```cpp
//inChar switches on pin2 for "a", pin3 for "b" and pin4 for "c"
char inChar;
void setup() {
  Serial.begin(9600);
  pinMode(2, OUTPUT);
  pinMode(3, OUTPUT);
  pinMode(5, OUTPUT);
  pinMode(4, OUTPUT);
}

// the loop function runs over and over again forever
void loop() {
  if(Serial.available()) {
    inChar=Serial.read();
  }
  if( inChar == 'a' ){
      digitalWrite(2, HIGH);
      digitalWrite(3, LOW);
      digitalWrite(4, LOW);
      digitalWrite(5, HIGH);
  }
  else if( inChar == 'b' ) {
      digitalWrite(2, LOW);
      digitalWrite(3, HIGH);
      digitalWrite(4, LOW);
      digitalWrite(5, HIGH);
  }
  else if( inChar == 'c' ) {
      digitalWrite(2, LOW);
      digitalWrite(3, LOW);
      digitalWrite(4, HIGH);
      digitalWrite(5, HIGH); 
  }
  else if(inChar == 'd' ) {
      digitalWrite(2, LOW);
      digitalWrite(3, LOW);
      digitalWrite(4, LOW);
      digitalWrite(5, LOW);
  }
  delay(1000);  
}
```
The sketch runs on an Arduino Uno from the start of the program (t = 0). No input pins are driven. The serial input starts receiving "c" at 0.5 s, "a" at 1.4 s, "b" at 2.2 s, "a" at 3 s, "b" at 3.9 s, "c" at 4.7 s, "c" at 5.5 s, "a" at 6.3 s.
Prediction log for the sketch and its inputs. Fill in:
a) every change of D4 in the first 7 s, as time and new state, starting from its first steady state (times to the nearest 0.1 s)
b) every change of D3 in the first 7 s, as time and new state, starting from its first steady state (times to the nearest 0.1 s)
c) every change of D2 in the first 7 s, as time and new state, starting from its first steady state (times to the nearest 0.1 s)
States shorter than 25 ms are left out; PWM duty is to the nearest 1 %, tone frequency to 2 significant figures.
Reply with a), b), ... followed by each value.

a) 0 s low; 1 s high; 2 s low; 6 s high
b) 0 s low; 3 s high; 4 s low; 5 s high; 6 s low
c) 0 s low; 2 s high; 3 s low; 4 s high; 5 s low
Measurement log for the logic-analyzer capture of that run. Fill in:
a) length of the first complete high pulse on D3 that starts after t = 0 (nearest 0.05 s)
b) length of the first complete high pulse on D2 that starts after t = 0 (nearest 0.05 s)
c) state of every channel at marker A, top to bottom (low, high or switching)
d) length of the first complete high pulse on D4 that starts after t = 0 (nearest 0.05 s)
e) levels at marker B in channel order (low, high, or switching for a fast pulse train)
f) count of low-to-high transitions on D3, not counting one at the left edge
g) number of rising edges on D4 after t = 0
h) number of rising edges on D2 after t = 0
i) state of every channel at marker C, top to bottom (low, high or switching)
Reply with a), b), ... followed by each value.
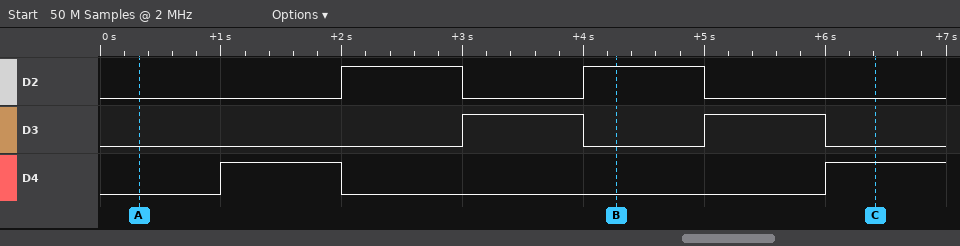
a) 1.00 s
b) 1.00 s
c) D2 low, D3 low, D4 low
d) 1.00 s
e) D2 high, D3 low, D4 low
f) 2
g) 2
h) 2
i) D2 low, D3 low, D4 high
